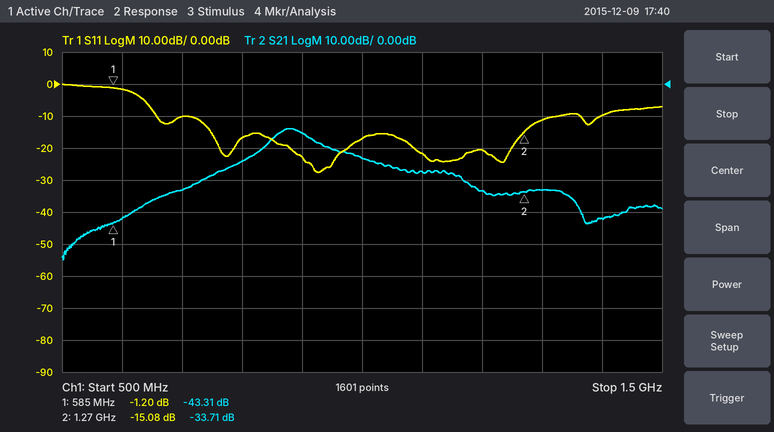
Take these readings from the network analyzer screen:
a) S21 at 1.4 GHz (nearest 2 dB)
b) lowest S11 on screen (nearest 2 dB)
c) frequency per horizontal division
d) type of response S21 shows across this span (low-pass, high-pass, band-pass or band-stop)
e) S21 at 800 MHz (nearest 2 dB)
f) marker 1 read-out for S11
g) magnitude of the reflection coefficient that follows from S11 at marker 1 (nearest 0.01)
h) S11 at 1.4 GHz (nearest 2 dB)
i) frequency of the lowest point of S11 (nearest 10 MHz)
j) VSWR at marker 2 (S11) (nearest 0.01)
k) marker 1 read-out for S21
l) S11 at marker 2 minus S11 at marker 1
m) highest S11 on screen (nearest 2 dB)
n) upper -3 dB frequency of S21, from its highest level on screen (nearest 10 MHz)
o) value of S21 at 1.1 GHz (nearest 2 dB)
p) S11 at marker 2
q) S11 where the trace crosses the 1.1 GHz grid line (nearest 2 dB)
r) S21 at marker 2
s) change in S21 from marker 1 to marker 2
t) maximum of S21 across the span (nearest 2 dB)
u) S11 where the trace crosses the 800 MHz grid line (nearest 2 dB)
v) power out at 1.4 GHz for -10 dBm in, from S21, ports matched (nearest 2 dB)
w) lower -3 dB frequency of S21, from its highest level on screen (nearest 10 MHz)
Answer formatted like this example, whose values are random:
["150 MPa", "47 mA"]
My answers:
["-42 dB", "-28 dB", "100 MHz", "band-pass", "-24 dB", "-1.20 dB", "0.87", "-10 dB", "930 MHz", "1.43", "-43.31 dB", "-13.88 dB", "0 dB", "910 MHz", "-28 dB", "-15.08 dB", "-22 dB", "-33.71 dB", "9.60 dB", "-14 dB", "-16 dB", "-52 dBm", "850 MHz"]
